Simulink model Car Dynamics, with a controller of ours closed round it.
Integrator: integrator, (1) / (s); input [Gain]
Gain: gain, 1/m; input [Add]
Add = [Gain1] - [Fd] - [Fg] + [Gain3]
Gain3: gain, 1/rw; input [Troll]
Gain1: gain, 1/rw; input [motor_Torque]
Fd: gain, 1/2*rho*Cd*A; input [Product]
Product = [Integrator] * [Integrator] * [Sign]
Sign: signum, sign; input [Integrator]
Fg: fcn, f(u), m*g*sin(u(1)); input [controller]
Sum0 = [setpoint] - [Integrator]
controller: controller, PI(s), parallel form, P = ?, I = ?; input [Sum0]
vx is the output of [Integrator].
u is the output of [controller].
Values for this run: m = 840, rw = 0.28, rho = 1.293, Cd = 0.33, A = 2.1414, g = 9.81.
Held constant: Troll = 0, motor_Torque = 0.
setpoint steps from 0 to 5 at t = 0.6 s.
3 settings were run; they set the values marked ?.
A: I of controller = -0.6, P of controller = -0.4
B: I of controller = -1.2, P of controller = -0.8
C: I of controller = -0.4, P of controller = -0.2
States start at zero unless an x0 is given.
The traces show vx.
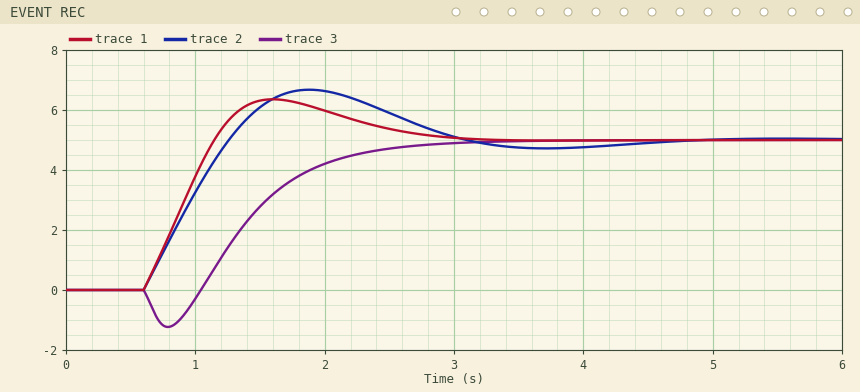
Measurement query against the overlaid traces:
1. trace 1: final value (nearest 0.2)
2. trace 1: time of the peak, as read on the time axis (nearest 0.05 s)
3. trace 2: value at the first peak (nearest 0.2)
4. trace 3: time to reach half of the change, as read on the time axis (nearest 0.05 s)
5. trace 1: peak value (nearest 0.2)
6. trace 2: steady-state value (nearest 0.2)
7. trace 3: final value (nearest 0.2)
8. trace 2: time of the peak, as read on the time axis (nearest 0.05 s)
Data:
5.0
1.60 s
6.6
1.45 s
6.4
5.0
5.0
1.90 s
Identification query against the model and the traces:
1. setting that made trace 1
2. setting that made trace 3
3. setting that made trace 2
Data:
A
B
C
